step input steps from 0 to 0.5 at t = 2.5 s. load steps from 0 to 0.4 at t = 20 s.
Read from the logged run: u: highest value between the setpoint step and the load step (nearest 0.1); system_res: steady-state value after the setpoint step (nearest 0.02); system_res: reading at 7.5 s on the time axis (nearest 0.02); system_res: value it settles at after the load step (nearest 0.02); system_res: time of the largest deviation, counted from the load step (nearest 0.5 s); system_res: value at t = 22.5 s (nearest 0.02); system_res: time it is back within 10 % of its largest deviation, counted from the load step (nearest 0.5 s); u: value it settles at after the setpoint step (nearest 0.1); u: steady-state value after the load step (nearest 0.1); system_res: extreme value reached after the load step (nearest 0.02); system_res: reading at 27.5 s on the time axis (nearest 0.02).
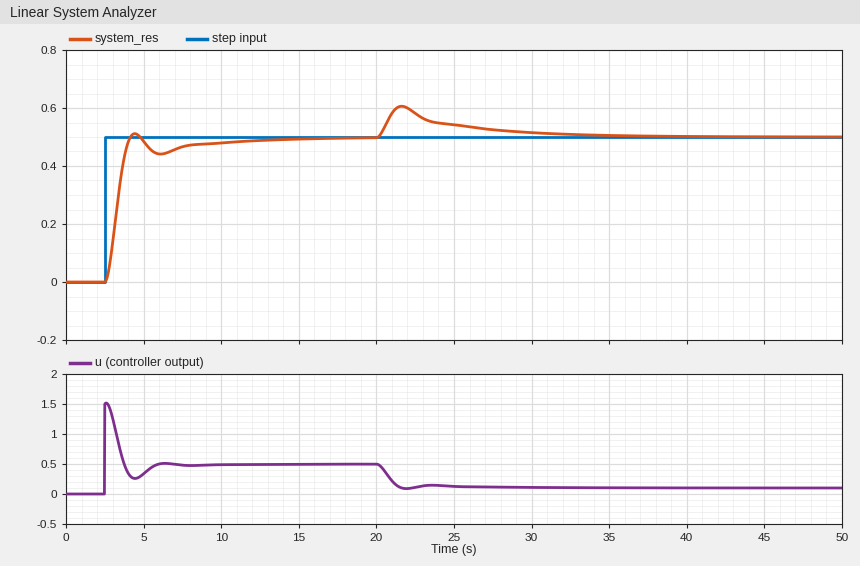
1.5
0.50
0.46
0.50
1.5 s
0.58
11.5 s
0.5
0.1
0.60
0.52
